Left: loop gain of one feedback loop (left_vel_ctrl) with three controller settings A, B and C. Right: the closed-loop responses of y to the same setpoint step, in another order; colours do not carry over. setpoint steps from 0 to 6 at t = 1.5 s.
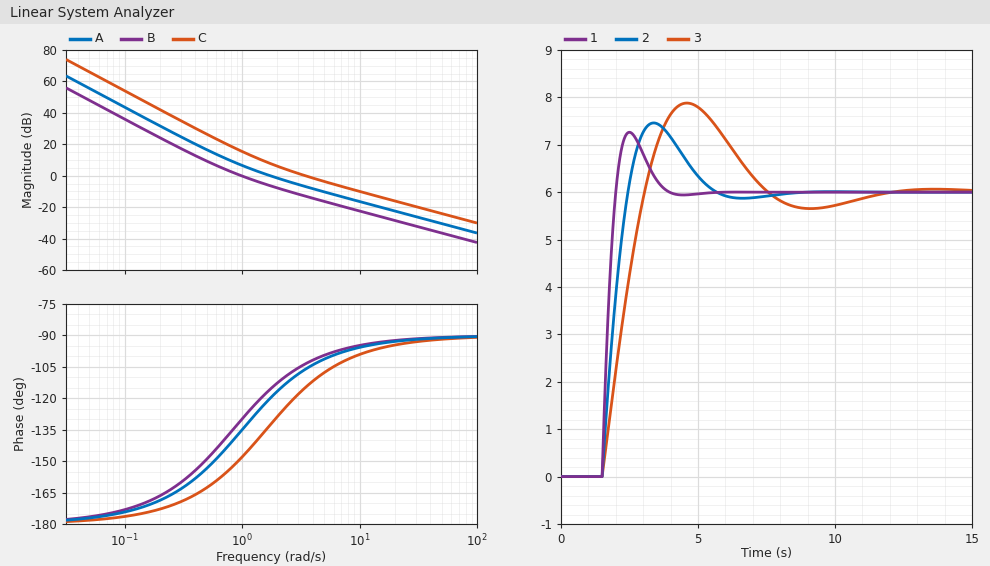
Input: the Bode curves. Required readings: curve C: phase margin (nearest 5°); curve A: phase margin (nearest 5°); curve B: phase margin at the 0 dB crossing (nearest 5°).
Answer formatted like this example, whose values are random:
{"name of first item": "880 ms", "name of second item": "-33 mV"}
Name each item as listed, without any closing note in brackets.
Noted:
{"curve C: phase margin": "65°", "curve A: phase margin": "60°", "curve B: phase margin at the 0 dB crossing": "50°"}
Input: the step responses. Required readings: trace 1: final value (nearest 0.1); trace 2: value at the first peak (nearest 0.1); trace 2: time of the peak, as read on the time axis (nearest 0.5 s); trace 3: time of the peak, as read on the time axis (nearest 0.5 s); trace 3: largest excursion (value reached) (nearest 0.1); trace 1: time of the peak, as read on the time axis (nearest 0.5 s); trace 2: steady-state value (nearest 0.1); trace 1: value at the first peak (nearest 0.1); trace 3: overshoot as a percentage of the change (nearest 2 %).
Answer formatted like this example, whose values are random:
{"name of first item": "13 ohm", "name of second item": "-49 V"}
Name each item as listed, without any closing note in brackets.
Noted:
{"trace 1: final value": "6.0", "trace 2: value at the first peak": "7.5", "trace 2: time of the peak, as read on the time axis": "3.5 s", "trace 3: time of the peak, as read on the time axis": "4.5 s", "trace 3: largest excursion (value reached)": "7.9", "trace 1: time of the peak, as read on the time axis": "2.5 s", "trace 2: steady-state value": "6.0", "trace 1: value at the first peak": "7.3", "trace 3: overshoot as a percentage of the change": "32 %"}
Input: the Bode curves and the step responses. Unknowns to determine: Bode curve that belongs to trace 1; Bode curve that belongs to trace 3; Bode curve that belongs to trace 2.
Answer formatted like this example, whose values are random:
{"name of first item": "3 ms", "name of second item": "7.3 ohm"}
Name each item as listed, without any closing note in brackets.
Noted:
{"Bode curve that belongs to trace 1": "C", "Bode curve that belongs to trace 3": "B", "Bode curve that belongs to trace 2": "A"}
